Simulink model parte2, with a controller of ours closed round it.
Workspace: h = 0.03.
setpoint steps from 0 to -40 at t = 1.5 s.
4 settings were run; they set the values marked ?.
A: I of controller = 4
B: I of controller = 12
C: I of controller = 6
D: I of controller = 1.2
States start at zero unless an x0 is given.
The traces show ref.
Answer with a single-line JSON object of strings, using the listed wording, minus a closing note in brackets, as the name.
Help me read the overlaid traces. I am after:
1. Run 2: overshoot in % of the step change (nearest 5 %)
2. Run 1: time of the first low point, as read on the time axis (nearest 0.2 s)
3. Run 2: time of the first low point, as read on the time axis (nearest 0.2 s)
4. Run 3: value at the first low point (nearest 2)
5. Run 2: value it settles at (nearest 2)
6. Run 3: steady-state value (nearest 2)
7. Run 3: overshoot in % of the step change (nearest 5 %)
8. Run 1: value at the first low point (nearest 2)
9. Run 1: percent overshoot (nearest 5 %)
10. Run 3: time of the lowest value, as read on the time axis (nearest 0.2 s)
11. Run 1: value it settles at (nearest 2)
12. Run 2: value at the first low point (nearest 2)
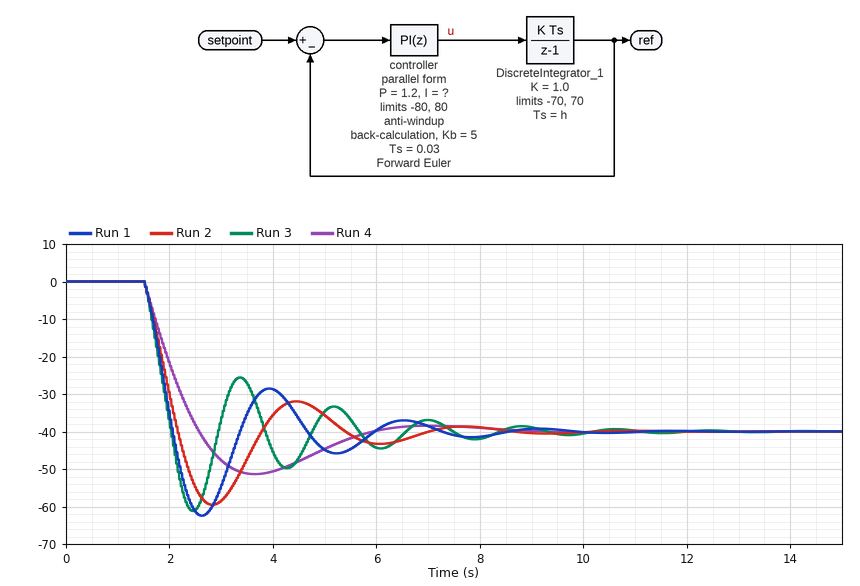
{"Run 2: overshoot in % of the step change": "50 %", "Run 1: time of the first low point, as read on the time axis": "2.6 s", "Run 2: time of the first low point, as read on the time axis": "2.8 s", "Run 3: value at the first low point": "-62", "Run 2: value it settles at": "-40", "Run 3: steady-state value": "-40", "Run 3: overshoot in % of the step change": "55 %", "Run 1: value at the first low point": "-62", "Run 1: percent overshoot": "55 %", "Run 3: time of the lowest value, as read on the time axis": "2.4 s", "Run 1: value it settles at": "-40", "Run 2: value at the first low point": "-60"}
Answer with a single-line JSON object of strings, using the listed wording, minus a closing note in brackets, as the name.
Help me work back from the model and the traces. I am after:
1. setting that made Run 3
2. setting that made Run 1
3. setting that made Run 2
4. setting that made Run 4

{"setting that made Run 3": "B", "setting that made Run 1": "C", "setting that made Run 2": "A", "setting that made Run 4": "D"}
